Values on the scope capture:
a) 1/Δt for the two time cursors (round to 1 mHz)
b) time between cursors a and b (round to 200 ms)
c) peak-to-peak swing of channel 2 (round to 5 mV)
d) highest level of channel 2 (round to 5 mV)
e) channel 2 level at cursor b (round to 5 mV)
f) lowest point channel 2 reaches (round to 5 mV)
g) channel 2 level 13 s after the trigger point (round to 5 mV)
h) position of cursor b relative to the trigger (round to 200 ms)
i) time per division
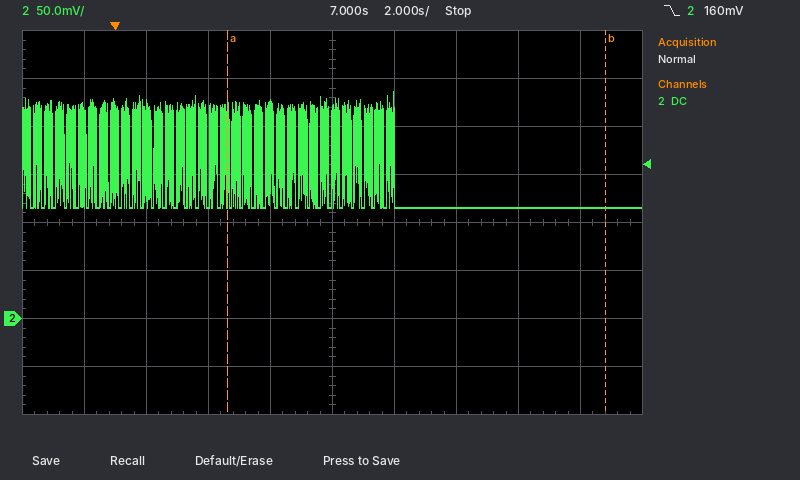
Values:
82 mHz
12.2 s
120 mV
235 mV
115 mV
115 mV
115 mV
+15.8 s
2 s
